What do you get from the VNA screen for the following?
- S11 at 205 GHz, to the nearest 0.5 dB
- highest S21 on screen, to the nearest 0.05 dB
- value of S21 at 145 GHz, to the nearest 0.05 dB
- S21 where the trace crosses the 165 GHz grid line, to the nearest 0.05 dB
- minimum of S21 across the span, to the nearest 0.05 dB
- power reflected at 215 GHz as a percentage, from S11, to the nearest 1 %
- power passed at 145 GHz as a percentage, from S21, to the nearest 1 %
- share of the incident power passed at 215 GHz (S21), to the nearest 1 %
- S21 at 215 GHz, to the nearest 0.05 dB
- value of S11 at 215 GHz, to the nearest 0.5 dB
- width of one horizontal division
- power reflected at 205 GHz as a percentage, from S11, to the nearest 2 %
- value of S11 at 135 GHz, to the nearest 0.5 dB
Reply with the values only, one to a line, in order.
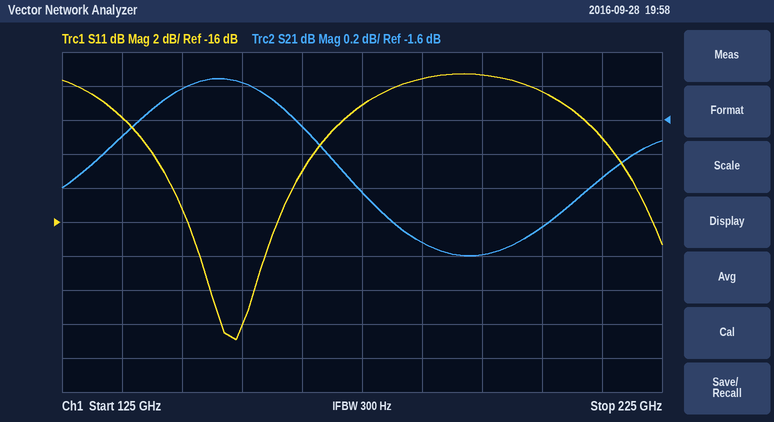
-8.5 dB
-1.35 dB
-1.40 dB
-1.65 dB
-2.40 dB
8 %
72 %
64 %
-1.95 dB
-11.0 dB
10 GHz
14 %
-10.0 dB
